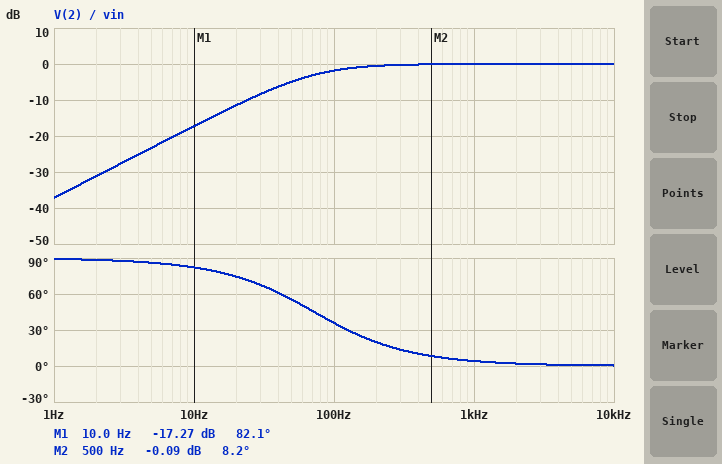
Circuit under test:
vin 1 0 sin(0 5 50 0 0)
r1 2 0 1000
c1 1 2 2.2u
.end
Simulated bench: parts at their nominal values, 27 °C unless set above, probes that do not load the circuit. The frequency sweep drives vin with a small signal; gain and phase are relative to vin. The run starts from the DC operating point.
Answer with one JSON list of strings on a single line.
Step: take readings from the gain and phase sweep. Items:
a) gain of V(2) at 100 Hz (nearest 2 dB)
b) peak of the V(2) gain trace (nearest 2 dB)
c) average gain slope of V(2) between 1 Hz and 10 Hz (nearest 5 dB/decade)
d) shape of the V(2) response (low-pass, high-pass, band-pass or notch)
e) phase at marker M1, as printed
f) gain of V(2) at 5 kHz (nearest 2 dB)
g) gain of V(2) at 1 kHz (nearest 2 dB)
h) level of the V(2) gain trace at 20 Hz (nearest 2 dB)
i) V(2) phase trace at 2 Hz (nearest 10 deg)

["-2 dB", "0 dB", "20 dB/decade", "high-pass", "82.1 deg", "0 dB", "0 dB", "-12 dB", "90 deg"]
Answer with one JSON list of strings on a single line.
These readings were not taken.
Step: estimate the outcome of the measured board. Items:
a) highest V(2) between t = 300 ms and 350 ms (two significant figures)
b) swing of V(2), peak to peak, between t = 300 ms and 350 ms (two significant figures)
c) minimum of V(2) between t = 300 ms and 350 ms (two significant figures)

["2.8 V", "5.7 V", "-2.8 V"]
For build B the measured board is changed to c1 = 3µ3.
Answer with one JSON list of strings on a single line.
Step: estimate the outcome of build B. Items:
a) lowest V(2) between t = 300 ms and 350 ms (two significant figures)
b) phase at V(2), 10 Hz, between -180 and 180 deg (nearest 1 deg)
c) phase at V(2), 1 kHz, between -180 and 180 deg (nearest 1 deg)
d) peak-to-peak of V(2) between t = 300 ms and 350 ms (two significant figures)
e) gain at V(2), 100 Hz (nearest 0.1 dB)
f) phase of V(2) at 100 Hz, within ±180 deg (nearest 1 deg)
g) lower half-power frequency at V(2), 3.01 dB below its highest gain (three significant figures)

["-3.6 V", "78 deg", "3 deg", "7.2 V", "-0.9 dB", "26 deg", "48.2 Hz"]
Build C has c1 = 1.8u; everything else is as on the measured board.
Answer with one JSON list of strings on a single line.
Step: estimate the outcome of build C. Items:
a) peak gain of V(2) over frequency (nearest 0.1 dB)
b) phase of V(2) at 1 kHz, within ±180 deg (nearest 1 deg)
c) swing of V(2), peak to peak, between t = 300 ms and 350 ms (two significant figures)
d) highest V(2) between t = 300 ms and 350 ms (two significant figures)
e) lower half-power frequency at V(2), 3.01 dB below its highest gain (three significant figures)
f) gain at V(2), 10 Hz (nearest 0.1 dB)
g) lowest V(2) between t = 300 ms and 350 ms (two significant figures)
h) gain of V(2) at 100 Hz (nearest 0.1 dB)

["0 dB", "5 deg", "4.9 V", "2.5 V", "88.4 Hz", "-19.0 dB", "-2.5 V", "-2.5 dB"]
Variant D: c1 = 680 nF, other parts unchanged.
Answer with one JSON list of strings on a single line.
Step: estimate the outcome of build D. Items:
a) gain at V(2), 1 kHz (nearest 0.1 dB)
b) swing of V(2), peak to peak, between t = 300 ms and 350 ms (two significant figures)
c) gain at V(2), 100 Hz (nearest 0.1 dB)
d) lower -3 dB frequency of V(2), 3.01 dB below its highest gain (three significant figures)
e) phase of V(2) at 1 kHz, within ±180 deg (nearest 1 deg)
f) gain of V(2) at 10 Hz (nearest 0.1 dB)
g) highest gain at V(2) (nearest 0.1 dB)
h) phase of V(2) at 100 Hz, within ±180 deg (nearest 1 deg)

["-0.2 dB", "2.1 V", "-8.1 dB", "234 Hz", "13 deg", "-27.4 dB", "0 dB", "67 deg"]
